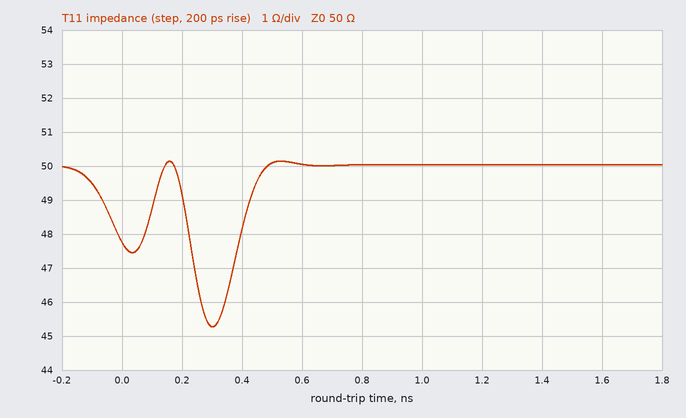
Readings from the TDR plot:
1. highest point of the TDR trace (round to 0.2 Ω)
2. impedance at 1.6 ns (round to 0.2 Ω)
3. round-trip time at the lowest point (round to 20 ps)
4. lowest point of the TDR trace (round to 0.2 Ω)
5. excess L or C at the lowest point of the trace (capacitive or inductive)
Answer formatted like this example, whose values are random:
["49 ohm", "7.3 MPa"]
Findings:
["50.2 Ω", "50.0 Ω", "300 ps", "45.2 Ω", "capacitive"]
